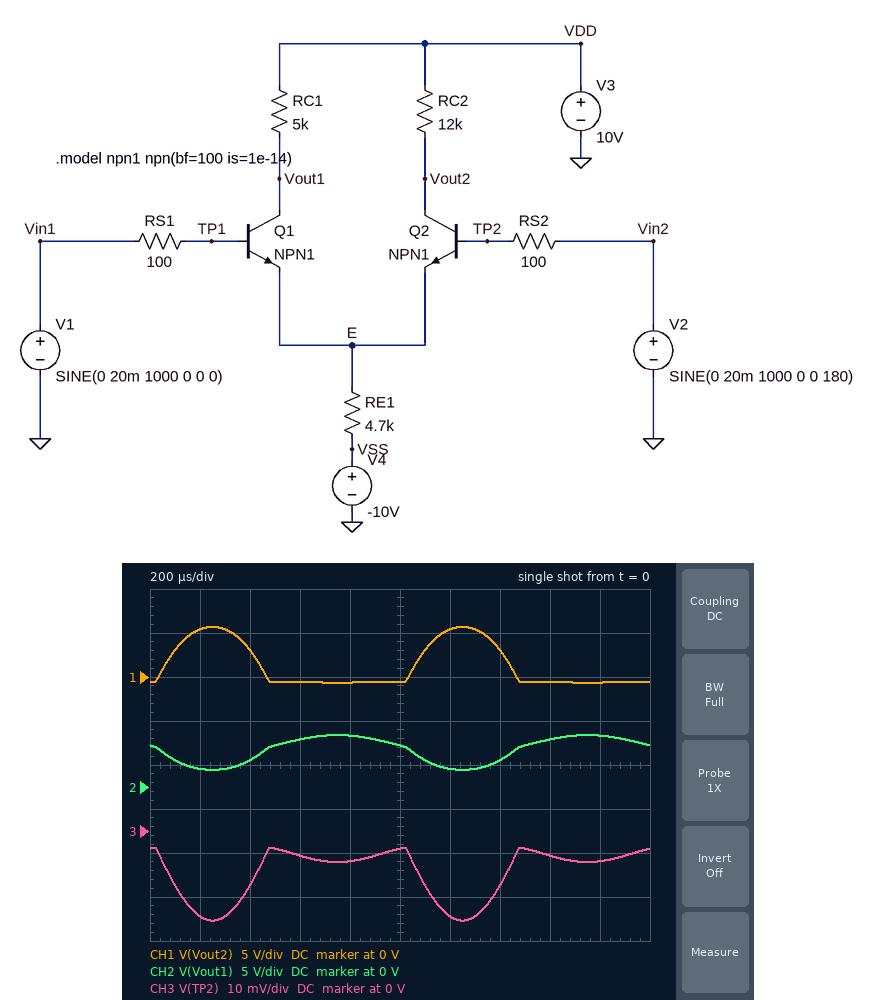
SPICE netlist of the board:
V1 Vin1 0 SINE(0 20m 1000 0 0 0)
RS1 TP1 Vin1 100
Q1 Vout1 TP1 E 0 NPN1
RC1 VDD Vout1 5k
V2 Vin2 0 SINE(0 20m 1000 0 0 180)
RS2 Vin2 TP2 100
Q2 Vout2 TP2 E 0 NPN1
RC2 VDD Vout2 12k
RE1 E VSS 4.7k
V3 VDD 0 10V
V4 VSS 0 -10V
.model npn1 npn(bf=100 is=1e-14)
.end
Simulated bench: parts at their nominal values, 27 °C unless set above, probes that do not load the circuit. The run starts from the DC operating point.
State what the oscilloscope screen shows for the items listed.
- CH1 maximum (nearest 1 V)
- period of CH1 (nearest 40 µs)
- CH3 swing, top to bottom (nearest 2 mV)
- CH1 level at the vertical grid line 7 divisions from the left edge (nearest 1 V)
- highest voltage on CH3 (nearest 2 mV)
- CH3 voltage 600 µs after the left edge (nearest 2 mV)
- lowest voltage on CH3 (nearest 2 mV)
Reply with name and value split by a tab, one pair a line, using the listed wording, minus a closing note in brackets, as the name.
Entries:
CH1 maximum	6 V
period of CH1	1.00 ms
CH3 swing, top to bottom	16 mV
CH1 level at the vertical grid line 7 divisions from the left edge	3 V
highest voltage on CH3	-4 mV
CH3 voltage 600 µs after the left edge	-6 mV
lowest voltage on CH3	-20 mV
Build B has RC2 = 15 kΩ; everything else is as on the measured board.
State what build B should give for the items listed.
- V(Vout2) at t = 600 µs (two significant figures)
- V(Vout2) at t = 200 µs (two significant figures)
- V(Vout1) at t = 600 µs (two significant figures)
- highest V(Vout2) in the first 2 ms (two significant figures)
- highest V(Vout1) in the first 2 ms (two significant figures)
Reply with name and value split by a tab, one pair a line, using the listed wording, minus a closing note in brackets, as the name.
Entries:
V(Vout2) at t = 600 µs	-630 mV
V(Vout2) at t = 200 µs	4.3 V
V(Vout1) at t = 600 µs	4.8 V
highest V(Vout2) in the first 2 ms	4.6 V
highest V(Vout1) in the first 2 ms	5.3 V
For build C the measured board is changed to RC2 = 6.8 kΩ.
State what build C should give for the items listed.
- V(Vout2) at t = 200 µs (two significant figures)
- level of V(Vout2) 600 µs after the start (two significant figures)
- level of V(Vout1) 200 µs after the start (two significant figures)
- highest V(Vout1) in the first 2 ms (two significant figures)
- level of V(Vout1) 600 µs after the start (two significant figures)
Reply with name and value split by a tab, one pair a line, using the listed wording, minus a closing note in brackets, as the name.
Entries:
V(Vout2) at t = 200 µs	7.4 V
level of V(Vout2) 600 µs after the start	540 mV
level of V(Vout1) 200 µs after the start	2.1 V
highest V(Vout1) in the first 2 ms	8.0 V
level of V(Vout1) 600 µs after the start	7.1 V
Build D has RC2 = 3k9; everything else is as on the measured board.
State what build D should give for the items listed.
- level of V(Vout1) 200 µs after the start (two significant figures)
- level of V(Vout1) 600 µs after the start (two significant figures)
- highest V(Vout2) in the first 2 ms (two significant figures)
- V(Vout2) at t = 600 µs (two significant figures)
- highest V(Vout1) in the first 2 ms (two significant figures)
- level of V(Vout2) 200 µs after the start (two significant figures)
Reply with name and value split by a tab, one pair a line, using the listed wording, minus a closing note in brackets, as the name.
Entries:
level of V(Vout1) 200 µs after the start	2.1 V
level of V(Vout1) 600 µs after the start	7.1 V
highest V(Vout2) in the first 2 ms	8.6 V
V(Vout2) at t = 600 µs	4.6 V
highest V(Vout1) in the first 2 ms	8.2 V
level of V(Vout2) 200 µs after the start	8.5 V
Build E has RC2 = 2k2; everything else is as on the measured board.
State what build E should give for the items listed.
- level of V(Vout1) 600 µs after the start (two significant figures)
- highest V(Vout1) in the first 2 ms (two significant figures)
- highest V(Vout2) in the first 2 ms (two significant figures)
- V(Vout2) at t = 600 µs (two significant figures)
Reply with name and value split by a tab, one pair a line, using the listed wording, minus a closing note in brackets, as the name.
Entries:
level of V(Vout1) 600 µs after the start	7.1 V
highest V(Vout1) in the first 2 ms	8.2 V
highest V(Vout2) in the first 2 ms	9.2 V
V(Vout2) at t = 600 µs	6.9 V
